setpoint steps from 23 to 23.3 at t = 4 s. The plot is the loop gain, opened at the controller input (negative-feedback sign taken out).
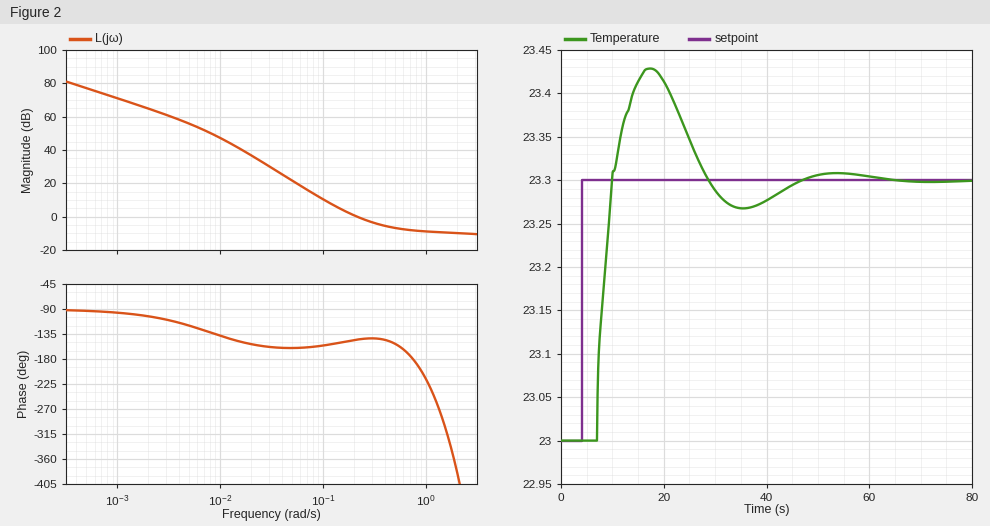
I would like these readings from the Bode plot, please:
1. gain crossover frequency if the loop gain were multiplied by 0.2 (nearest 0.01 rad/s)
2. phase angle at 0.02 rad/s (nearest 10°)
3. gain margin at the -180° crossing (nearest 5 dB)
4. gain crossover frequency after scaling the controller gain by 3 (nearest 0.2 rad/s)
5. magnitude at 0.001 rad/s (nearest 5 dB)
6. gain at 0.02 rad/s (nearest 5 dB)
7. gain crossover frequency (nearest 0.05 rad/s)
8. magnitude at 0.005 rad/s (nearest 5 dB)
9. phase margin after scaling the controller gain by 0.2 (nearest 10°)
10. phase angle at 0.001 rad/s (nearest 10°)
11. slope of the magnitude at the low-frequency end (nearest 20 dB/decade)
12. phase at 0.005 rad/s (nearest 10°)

0.08 rad/s
-150°
10 dB
1.6 rad/s
70 dB
35 dB
0.20 rad/s
55 dB
20°
-100°
-20 dB/decade
-120°
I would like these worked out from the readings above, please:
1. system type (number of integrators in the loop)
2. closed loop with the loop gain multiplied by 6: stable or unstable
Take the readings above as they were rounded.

1
unstable
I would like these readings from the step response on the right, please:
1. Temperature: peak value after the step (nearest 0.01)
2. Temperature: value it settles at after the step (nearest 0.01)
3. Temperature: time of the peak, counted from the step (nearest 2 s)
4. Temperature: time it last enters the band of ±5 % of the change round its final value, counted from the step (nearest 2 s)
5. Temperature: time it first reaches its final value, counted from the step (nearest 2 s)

23.43
23.30
14 s
38 s
6 s
